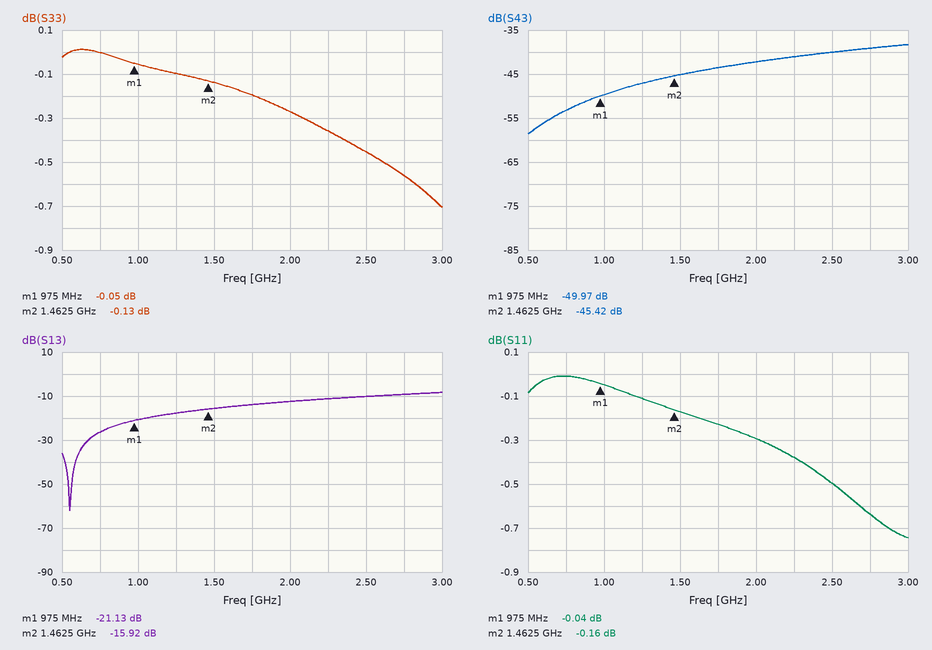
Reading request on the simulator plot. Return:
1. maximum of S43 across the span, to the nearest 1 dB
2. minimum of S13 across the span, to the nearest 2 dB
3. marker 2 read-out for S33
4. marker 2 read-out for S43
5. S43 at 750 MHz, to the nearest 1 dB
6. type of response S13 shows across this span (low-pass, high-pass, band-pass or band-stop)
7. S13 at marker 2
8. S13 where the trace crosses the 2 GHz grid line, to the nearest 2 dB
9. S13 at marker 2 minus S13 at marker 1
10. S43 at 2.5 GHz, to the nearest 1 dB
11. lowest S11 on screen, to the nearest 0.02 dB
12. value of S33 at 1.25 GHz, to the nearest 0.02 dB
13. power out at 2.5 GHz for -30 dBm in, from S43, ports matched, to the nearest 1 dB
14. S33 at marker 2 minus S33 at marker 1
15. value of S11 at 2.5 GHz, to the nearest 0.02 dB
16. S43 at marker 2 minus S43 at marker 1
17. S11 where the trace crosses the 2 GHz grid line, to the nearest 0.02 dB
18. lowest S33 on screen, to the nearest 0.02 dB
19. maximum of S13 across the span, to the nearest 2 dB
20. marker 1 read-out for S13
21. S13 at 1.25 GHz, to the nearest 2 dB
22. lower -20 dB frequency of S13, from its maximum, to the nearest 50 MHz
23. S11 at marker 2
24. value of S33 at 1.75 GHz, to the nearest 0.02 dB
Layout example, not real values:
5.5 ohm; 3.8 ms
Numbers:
-38 dB; -62 dB; -0.13 dB; -45.42 dB; -53 dB; high-pass; -15.92 dB; -12 dB; 5.21 dB; -40 dB; -0.74 dB; -0.10 dB; -70 dBm; -0.08 dB; -0.50 dB; 4.55 dB; -0.30 dB; -0.70 dB; -8 dB; -21.13 dB; -18 dB; 700 MHz; -0.16 dB; -0.20 dB
